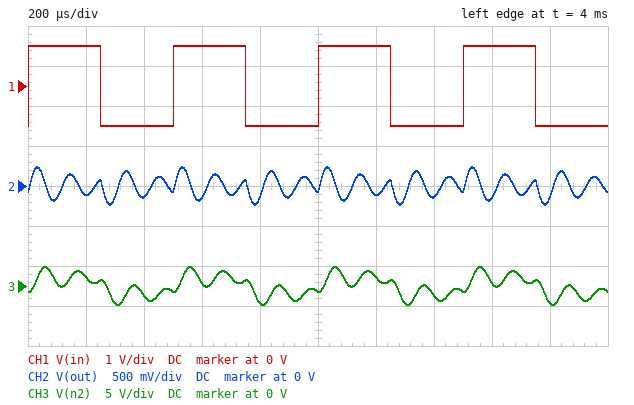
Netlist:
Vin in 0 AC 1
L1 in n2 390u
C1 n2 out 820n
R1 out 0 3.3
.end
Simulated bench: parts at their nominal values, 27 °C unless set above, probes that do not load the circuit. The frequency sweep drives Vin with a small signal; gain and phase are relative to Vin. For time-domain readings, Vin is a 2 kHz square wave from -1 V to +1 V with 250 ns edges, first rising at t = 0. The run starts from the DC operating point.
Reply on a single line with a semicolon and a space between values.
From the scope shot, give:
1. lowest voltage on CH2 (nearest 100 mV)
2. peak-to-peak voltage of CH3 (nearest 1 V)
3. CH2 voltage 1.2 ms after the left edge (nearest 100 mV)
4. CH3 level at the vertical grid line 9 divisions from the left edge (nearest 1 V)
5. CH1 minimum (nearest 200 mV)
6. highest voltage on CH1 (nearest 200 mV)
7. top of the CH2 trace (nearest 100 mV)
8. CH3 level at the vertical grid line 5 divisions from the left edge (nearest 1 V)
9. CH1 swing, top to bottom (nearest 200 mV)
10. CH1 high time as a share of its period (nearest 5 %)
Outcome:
-200 mV; 5 V; -100 mV; -2 V; -1.0 V; 1.0 V; 200 mV; -1 V; 2.0 V; 50 %
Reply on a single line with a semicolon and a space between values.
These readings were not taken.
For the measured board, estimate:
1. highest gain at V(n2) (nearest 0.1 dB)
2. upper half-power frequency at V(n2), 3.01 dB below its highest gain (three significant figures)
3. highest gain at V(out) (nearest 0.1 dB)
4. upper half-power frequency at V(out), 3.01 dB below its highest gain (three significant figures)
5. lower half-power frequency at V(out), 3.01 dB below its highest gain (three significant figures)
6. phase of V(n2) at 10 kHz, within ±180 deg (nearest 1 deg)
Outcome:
16.5 dB; 9.50 kHz; 0 dB; 9.60 kHz; 8.25 kHz; -137 deg
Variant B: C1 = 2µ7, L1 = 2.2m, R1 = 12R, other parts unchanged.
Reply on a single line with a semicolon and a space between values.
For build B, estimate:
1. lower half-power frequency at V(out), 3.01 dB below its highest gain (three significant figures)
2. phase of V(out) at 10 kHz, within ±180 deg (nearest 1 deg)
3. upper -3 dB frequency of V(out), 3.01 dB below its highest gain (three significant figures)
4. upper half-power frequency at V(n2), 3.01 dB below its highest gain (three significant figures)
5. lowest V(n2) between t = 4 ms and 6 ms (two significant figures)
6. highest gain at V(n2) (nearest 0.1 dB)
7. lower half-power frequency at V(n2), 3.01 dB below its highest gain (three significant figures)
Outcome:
1.68 kHz; -85 deg; 2.54 kHz; 2.40 kHz; -3.3 V; 8.4 dB; 1.50 kHz
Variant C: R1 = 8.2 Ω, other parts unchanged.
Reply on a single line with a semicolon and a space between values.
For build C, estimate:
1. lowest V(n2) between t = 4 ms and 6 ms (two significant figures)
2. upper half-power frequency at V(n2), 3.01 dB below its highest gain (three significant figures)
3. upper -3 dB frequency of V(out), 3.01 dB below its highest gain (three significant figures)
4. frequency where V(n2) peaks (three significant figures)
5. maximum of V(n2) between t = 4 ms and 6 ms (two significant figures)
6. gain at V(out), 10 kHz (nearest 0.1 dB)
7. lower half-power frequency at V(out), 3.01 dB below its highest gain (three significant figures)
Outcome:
-2.1 V; 10.2 kHz; 10.7 kHz; 8.62 kHz; 2.1 V; -1.4 dB; 7.38 kHz
